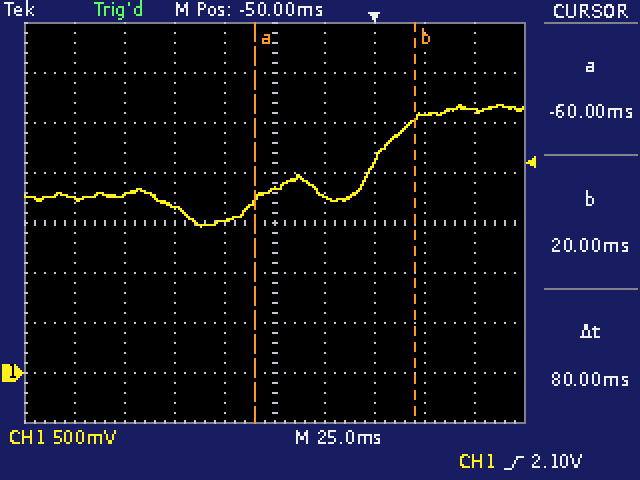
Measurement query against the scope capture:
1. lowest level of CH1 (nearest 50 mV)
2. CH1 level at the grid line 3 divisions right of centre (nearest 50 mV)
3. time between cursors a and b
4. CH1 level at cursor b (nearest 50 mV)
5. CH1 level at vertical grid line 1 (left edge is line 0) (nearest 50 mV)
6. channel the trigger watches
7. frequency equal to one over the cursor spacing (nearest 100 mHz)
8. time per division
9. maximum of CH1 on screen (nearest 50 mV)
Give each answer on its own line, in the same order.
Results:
1.45 V
2.60 V
80 ms
2.55 V
1.75 V
CH1
12.5 Hz
25 ms
2.70 V
